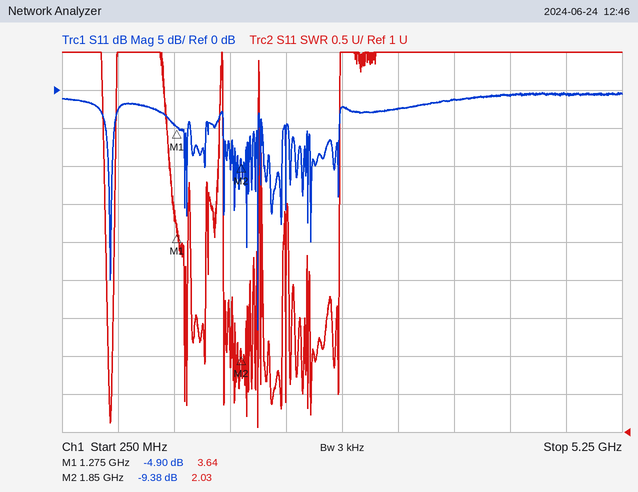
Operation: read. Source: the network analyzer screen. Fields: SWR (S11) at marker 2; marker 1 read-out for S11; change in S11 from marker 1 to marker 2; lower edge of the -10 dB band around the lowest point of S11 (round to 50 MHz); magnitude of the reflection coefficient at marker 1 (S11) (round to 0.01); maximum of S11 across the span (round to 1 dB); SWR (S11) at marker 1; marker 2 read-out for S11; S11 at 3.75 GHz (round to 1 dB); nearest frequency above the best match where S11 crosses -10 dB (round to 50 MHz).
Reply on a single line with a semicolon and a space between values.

2.03; -4.90 dB; -4.48 dB; 2.00 GHz; 0.57; 0 dB; 3.64; -9.38 dB; -1 dB; 2.00 GHz
